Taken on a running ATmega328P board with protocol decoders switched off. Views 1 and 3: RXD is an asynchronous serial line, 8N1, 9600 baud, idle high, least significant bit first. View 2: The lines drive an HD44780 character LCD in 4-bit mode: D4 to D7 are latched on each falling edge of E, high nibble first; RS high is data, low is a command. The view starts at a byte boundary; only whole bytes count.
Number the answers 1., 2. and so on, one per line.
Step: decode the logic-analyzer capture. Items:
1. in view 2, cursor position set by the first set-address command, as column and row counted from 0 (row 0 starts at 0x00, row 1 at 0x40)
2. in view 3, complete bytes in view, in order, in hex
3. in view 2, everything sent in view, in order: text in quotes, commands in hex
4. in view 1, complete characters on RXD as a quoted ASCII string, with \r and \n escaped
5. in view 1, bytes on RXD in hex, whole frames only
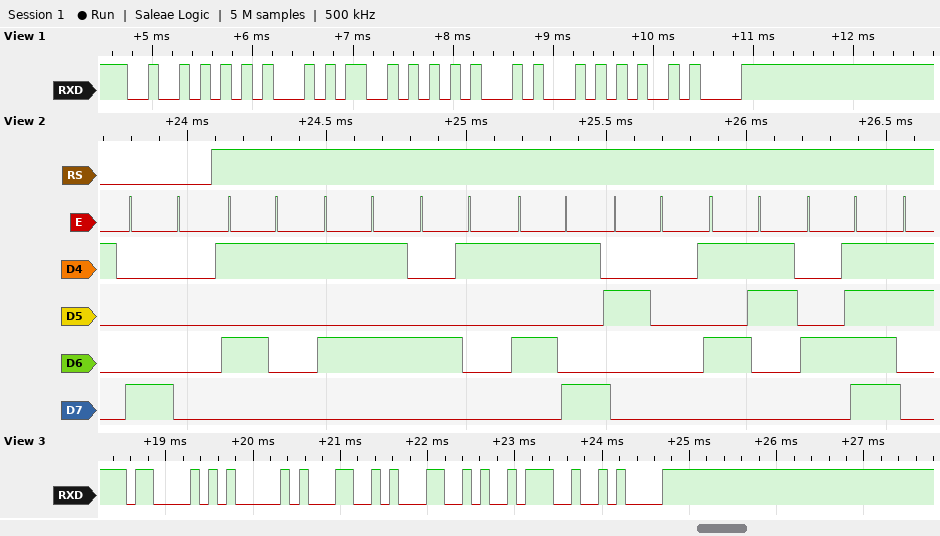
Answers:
1. column 0, row 0
2. 43 41 4C 4C 3A 0A
3. 0x80 "QUAY SO"
4. "RESET\n"
5. 0x52 0x45 0x53 0x45 0x54 0x0A
